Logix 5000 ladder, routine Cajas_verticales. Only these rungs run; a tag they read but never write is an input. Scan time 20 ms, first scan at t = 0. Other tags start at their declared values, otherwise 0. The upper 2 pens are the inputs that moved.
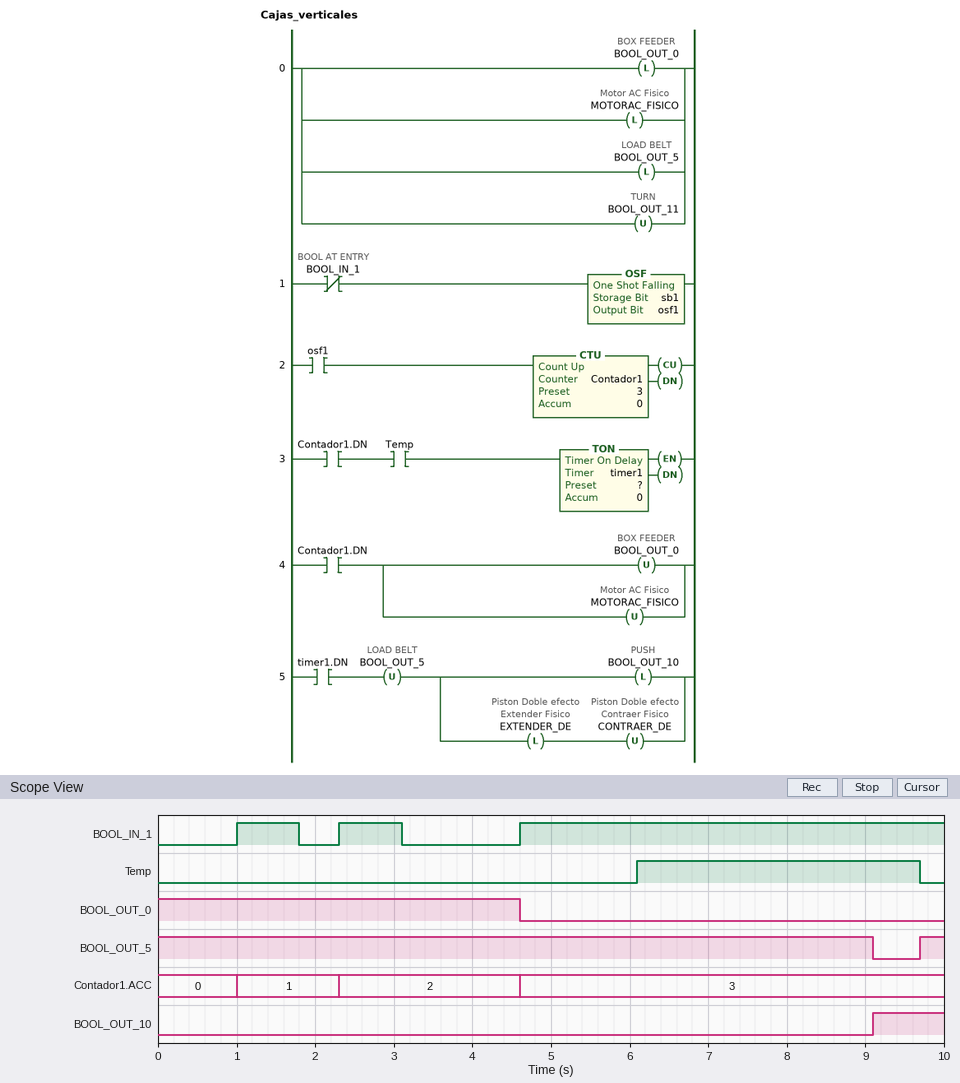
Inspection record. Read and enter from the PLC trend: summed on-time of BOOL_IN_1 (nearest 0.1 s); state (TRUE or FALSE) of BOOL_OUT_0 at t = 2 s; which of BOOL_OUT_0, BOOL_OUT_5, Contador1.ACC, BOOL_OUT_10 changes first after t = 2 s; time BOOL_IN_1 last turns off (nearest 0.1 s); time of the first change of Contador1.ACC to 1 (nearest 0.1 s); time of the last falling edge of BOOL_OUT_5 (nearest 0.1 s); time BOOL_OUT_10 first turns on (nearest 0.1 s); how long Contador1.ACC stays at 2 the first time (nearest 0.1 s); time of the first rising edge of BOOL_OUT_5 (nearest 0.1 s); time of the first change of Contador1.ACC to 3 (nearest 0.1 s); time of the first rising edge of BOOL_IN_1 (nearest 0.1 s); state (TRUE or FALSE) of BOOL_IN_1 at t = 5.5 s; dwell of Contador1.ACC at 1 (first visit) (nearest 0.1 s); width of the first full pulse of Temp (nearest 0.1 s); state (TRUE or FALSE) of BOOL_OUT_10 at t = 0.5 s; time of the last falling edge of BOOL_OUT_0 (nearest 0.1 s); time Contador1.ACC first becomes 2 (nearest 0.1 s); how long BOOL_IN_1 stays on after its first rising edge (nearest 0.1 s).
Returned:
7.0 s
TRUE
Contador1.ACC
3.1 s
1.0 s
9.1 s
9.1 s
2.3 s
9.7 s
4.6 s
1.0 s
TRUE
1.3 s
3.6 s
FALSE
4.6 s
2.3 s
0.8 s
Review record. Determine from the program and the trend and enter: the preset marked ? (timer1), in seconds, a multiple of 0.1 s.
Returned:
3.0 s
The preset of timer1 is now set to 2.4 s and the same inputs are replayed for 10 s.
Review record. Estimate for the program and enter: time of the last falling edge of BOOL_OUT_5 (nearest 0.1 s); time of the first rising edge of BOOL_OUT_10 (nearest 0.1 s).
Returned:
8.5 s
8.5 s
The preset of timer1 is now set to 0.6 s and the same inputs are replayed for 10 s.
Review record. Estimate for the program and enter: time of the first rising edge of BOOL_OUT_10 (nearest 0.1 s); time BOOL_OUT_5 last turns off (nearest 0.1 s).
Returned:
6.7 s
6.7 s
